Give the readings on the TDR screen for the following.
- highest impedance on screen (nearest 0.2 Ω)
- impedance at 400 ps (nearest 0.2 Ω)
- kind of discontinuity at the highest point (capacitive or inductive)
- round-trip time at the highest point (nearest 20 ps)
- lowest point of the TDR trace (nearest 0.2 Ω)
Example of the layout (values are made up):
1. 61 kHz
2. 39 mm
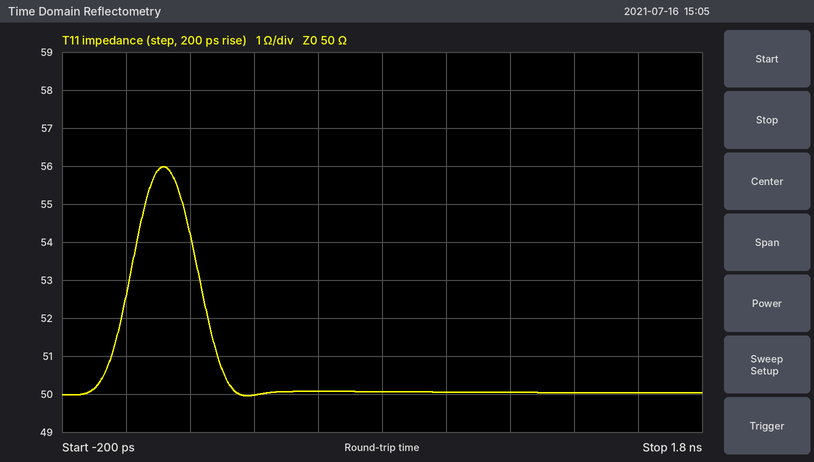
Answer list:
1. 56.0 Ω
2. 50.0 Ω
3. inductive
4. 120 ps
5. 50.0 Ω
